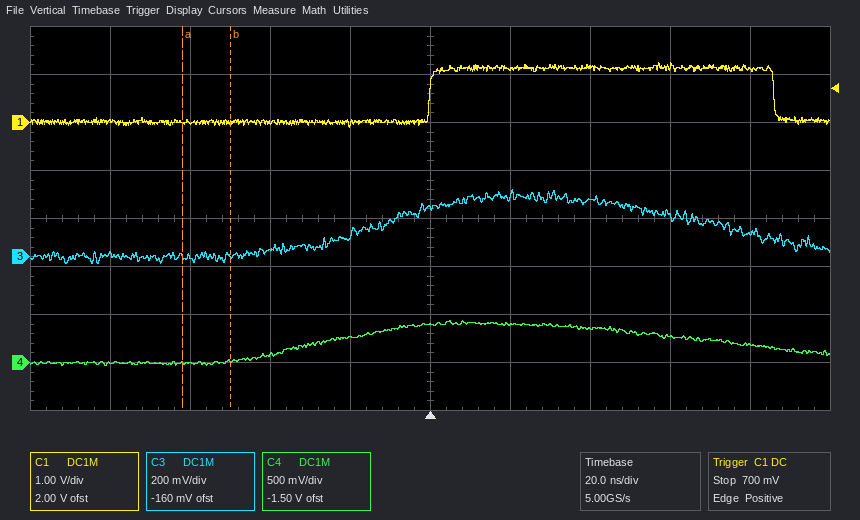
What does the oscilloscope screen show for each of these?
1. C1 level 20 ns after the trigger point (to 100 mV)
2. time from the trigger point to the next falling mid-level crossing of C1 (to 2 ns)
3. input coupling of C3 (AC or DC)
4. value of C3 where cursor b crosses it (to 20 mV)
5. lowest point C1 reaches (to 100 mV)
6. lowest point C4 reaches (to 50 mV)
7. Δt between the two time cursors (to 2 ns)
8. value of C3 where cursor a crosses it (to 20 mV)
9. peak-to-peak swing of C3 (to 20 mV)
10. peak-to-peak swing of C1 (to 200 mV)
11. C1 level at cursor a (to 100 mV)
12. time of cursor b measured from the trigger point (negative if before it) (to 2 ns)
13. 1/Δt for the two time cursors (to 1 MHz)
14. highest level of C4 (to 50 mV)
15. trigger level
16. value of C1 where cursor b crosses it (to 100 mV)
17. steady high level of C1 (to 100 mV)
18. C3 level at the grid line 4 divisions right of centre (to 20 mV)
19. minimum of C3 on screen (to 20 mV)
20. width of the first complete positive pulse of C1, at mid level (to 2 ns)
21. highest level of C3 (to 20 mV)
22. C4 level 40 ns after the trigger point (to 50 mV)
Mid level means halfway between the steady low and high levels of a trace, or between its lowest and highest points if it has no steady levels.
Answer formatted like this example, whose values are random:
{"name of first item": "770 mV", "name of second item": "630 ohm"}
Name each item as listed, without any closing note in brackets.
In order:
{"C1 level 20 ns after the trigger point": "1.1 V", "time from the trigger point to the next falling mid-level crossing of C1": "86 ns", "input coupling of C3": "DC", "value of C3 where cursor b crosses it": "0 mV", "lowest point C1 reaches": "-100 mV", "lowest point C4 reaches": "-50 mV", "Δt between the two time cursors": "12 ns", "value of C3 where cursor a crosses it": "0 mV", "peak-to-peak swing of C3": "300 mV", "peak-to-peak swing of C1": "1.4 V", "C1 level at cursor a": "0.0 V", "time of cursor b measured from the trigger point (negative if before it)": "-50 ns", "1/Δt for the two time cursors": "83 MHz", "highest level of C4": "450 mV", "trigger level": "700 mV", "value of C1 where cursor b crosses it": "0.0 V", "steady high level of C1": "1.1 V", "C3 level at the grid line 4 divisions right of centre": "100 mV", "minimum of C3 on screen": "-20 mV", "width of the first complete positive pulse of C1, at mid level": "86 ns", "highest level of C3": "280 mV", "C4 level 40 ns after the trigger point": "350 mV"}
